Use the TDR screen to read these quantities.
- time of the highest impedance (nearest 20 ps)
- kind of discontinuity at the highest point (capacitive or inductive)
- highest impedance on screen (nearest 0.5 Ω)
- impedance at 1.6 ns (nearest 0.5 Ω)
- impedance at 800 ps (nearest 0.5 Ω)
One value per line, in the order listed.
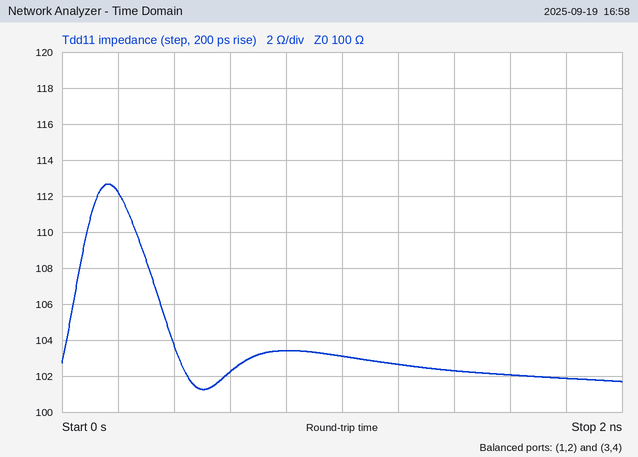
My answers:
160 ps
inductive
112.5 Ω
102.0 Ω
103.5 Ω
